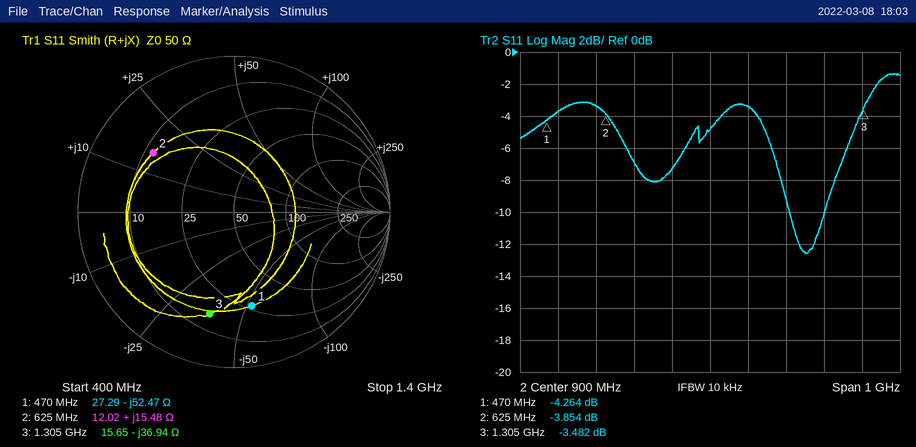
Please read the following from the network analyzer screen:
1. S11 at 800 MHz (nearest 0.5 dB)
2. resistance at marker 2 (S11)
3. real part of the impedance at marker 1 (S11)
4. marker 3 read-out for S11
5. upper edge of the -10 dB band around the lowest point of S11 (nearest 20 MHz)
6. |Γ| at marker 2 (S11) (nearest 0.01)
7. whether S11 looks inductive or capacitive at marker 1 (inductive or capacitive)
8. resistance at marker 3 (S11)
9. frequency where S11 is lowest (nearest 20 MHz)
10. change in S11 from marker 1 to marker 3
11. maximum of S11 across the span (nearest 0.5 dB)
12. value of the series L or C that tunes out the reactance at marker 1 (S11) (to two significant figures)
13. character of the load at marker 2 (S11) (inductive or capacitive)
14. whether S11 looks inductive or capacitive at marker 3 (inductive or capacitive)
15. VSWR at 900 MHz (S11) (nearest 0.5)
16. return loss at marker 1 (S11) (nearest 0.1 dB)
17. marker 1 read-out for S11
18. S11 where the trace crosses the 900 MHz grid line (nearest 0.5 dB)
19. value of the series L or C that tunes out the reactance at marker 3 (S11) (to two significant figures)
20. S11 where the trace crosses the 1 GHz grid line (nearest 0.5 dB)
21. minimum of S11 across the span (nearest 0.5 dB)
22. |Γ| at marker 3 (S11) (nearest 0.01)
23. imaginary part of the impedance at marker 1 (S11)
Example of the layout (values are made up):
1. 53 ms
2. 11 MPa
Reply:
1. -7.5 dB
2. 12.02 Ω
3. 27.29 Ω
4. -3.482 dB
5. 1.20 GHz
6. 0.64
7. capacitive
8. 15.65 Ω
9. 1.16 GHz
10. 0.782 dB
11. -1.5 dB
12. 18 nH
13. inductive
14. capacitive
15. 3.5
16. 4.3 dB
17. -4.264 dB
18. -5.0 dB
19. 4.5 nH
20. -3.5 dB
21. -12.5 dB
22. 0.67
23. -52.47 Ω
